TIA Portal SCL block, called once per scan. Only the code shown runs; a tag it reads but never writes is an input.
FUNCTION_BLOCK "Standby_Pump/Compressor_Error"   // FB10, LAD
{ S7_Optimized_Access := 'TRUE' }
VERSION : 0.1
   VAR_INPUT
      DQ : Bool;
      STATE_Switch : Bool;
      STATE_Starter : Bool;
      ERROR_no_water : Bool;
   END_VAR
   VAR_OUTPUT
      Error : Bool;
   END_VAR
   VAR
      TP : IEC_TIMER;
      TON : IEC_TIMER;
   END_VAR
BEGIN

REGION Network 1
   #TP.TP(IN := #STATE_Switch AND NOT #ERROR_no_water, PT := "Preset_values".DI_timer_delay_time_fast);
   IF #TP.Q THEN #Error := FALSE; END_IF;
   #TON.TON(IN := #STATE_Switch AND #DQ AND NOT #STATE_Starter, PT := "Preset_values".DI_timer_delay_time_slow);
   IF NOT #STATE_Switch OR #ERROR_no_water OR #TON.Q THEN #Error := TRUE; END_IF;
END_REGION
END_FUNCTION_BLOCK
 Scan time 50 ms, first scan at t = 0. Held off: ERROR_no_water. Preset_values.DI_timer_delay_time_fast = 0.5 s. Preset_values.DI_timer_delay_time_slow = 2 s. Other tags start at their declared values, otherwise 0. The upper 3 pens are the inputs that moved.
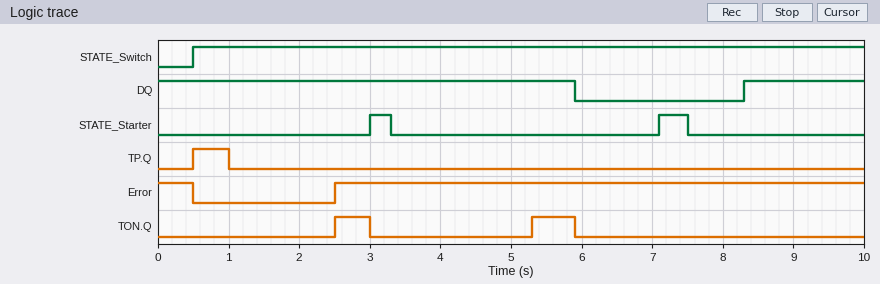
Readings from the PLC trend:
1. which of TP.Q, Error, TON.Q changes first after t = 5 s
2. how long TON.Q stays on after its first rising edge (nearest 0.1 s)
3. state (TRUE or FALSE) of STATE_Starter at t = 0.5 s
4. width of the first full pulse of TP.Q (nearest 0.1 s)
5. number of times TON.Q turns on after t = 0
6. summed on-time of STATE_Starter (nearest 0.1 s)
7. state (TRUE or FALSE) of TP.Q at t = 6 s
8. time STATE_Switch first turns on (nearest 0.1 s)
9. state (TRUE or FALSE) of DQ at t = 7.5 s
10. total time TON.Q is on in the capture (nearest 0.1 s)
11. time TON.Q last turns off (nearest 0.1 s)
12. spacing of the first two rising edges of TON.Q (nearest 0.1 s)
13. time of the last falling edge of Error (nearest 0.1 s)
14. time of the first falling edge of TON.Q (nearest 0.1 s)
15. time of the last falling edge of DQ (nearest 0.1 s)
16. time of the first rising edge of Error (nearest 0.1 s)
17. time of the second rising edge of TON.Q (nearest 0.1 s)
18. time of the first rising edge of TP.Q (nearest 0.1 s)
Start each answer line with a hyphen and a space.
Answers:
- TON.Q
- 0.5 s
- FALSE
- 0.5 s
- 2
- 0.7 s
- FALSE
- 0.5 s
- FALSE
- 1.1 s
- 5.9 s
- 2.8 s
- 0.5 s
- 3.0 s
- 5.9 s
- 2.5 s
- 5.3 s
- 0.5 s
